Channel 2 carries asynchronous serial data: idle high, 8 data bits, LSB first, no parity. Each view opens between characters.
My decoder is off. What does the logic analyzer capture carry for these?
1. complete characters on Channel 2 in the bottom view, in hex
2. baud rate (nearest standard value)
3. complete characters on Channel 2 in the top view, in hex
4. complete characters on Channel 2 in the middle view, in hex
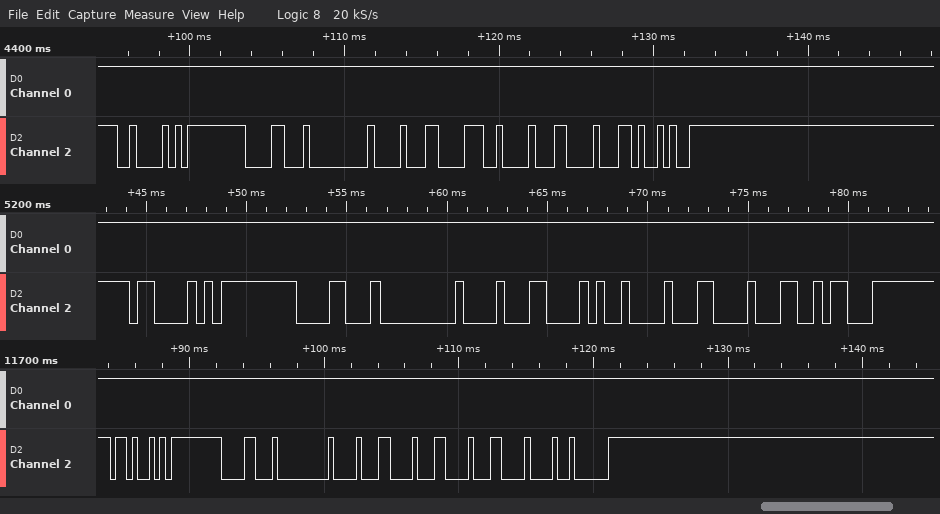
4B, FF, 18, 00, 88, 88, 88, 08, 02
2400 baud
42, FF, 18, 00, 88, 38, 88, 88, 29
43, FF, 18, 00, 88, 28, 88, 88, 1A
